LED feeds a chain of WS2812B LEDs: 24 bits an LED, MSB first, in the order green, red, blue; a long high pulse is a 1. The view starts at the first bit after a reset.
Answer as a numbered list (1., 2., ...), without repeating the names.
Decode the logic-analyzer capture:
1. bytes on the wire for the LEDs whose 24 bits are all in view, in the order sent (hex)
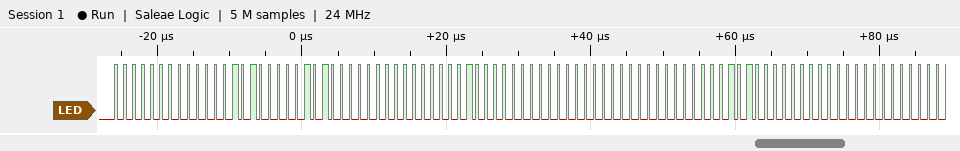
1. 00 05 05 00 01 00 00 00 0A
